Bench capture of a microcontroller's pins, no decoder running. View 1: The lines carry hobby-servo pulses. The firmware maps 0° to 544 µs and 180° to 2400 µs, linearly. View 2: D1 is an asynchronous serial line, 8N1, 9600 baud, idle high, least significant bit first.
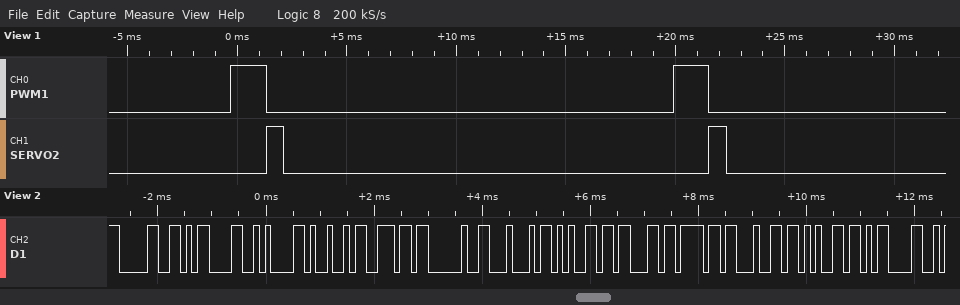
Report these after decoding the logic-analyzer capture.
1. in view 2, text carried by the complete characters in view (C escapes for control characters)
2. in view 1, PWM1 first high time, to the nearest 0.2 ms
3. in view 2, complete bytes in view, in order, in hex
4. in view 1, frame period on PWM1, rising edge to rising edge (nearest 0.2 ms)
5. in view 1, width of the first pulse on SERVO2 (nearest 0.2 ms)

"0\r\nIn Decode\r"
1.6 ms
30 0D 0A 49 6E 20 44 65 63 6F 64 65 0D
20.2 ms
0.8 ms
